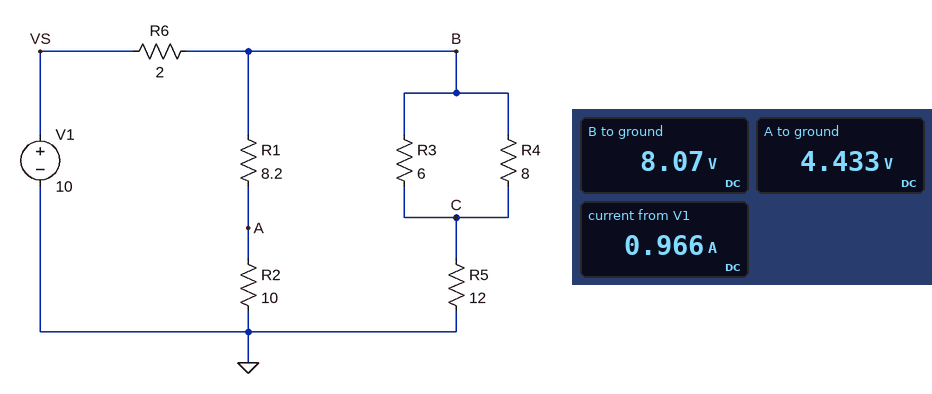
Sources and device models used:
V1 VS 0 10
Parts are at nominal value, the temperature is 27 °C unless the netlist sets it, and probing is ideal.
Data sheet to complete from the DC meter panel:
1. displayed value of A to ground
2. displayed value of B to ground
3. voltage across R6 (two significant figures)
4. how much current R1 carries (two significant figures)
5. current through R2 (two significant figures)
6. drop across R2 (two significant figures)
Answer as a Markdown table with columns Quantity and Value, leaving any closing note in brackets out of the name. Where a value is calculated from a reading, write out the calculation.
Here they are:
| Quantity | Value |
|---|---|
| displayed value of A to ground | 4.433 V |
| displayed value of B to ground | 8.07 V |
| voltage across R6 | 10 V - 8.07 V = 1.9 V |
| how much current R1 carries | (8.07 V - 4.433 V) / 8.2 Ω = 440 mA |
| current through R2 | (4.433 V) / 10 Ω = 440 mA |
| drop across R2 | 4.433 V = 4.4 V |
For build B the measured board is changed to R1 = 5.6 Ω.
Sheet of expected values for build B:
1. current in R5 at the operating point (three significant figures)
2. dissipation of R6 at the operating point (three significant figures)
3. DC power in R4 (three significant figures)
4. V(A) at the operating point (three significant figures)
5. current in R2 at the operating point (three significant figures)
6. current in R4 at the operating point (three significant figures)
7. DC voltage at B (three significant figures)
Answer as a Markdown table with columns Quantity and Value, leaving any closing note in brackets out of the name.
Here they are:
| Quantity | Value |
|---|---|
| current in R5 at the operating point | 515 mA |
| dissipation of R6 at the operating point | 2.10 W |
| DC power in R4 | 390 mW |
| V(A) at the operating point | 5.10 V |
| current in R2 at the operating point | 510 mA |
| current in R4 at the operating point | 221 mA |
| DC voltage at B | 7.95 V |
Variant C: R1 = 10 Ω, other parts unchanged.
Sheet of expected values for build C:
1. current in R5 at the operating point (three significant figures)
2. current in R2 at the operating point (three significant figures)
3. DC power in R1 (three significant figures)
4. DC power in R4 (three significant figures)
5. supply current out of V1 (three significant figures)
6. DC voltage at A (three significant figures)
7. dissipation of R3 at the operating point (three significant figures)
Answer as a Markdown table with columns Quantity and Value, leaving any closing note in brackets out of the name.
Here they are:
| Quantity | Value |
|---|---|
| current in R5 at the operating point | 527 mA |
| current in R2 at the operating point | 407 mA |
| DC power in R1 | 1.65 W |
| DC power in R4 | 408 mW |
| supply current out of V1 | 934 mA |
| DC voltage at A | 4.07 V |
| dissipation of R3 at the operating point | 544 mW |
